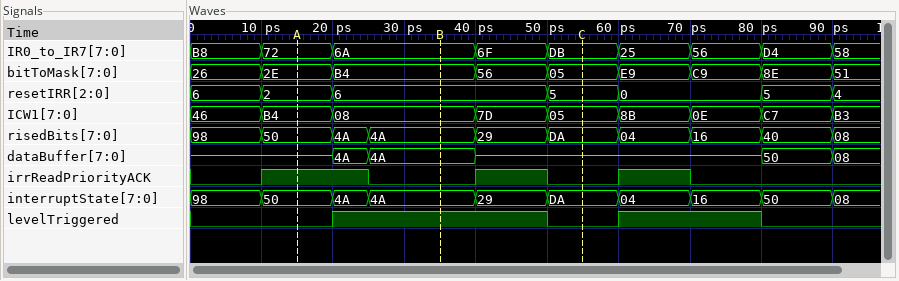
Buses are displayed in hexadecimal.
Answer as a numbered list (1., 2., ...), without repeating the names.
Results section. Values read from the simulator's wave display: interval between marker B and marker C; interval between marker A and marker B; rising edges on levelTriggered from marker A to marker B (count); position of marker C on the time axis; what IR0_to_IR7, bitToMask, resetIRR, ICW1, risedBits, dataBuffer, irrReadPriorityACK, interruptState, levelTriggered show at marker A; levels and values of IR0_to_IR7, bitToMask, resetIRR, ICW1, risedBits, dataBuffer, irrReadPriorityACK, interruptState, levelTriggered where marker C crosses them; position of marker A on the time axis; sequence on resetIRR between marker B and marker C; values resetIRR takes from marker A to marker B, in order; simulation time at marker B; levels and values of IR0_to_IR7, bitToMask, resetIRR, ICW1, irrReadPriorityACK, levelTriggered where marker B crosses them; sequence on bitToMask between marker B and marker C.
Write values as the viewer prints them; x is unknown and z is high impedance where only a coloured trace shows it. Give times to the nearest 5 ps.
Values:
1. 20 ps
2. 20 ps
3. 1
4. 55 ps
5. IR0_to_IR7=72, bitToMask=2E, resetIRR=2, ICW1=B4, risedBits=50, dataBuffer=z, irrReadPriorityACK=1, interruptState=50, levelTriggered=0
6. IR0_to_IR7=DB, bitToMask=05, resetIRR=5, ICW1=05, risedBits=DA, dataBuffer=z, irrReadPriorityACK=0, interruptState=DA, levelTriggered=0
7. 15 ps
8. 6, 5
9. 2, 6
10. 35 ps
11. IR0_to_IR7=6A, bitToMask=B4, resetIRR=6, ICW1=08, irrReadPriorityACK=0, levelTriggered=1
12. B4, 56, 05
